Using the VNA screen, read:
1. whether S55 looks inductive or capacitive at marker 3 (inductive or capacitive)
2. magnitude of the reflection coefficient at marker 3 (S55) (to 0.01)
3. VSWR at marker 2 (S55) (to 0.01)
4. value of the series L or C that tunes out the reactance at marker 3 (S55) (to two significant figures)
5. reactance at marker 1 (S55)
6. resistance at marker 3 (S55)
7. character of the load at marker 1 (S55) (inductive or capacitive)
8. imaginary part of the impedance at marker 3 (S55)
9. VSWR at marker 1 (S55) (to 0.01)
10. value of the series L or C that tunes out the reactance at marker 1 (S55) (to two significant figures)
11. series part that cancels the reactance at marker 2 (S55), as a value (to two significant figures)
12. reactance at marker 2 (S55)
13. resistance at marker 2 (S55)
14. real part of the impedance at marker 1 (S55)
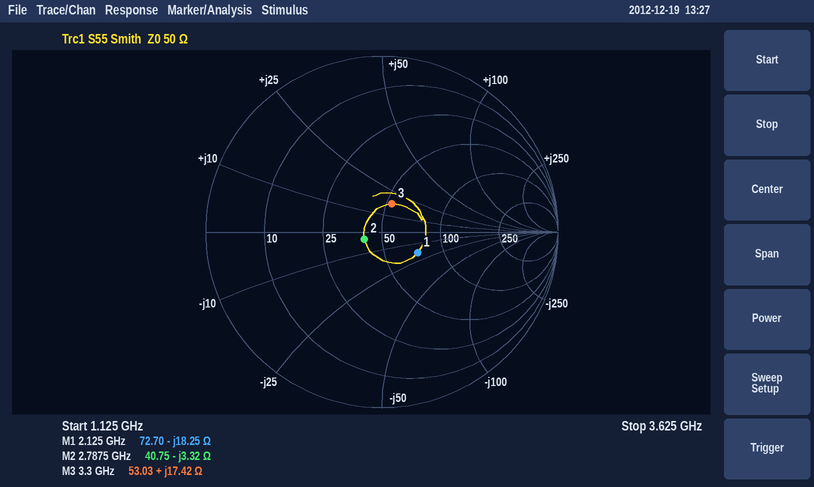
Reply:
inductive
0.17
1.24
2.8 pF
-18.25 Ω
53.03 Ω
capacitive
+17.42 Ω
1.61
1.4 nH
190 pH
-3.32 Ω
40.75 Ω
72.70 Ω
